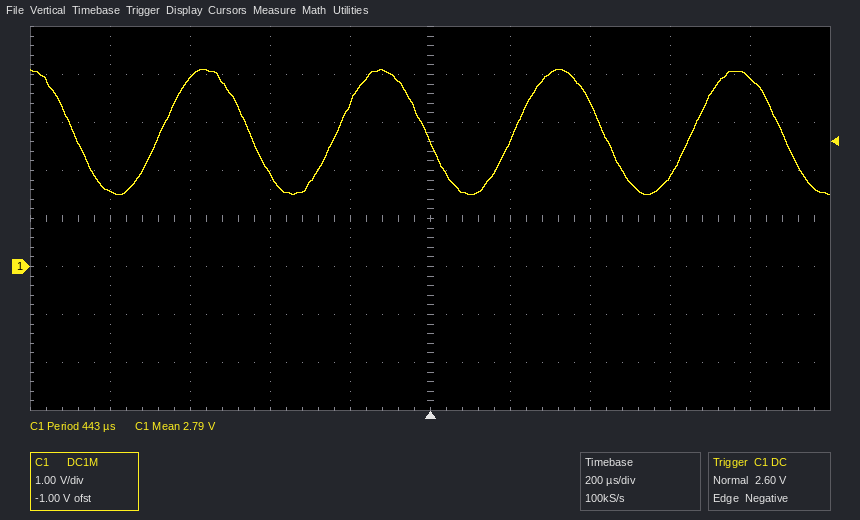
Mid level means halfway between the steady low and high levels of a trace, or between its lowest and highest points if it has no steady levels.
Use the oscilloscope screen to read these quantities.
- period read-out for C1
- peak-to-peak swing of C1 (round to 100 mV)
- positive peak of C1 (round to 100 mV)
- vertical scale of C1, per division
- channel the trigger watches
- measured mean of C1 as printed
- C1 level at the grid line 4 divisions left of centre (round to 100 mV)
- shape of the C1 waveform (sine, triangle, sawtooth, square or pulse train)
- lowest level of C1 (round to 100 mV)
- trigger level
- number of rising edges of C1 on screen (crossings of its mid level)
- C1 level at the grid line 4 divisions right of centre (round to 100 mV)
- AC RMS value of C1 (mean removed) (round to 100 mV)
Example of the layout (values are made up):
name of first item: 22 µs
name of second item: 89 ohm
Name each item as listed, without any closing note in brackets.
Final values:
period read-out for C1: 443 µs
peak-to-peak swing of C1: 2.6 V
positive peak of C1: 4.1 V
vertical scale of C1, per division: 1 V
channel the trigger watches: C1
measured mean of C1 as printed: 2.79 V
C1 level at the grid line 4 divisions left of centre: 1.6 V
shape of the C1 waveform: sine
lowest level of C1: 1.5 V
trigger level: 2.60 V
number of rising edges of C1 on screen: 4
C1 level at the grid line 4 divisions right of centre: 3.9 V
AC RMS value of C1 (mean removed): 900 mV
